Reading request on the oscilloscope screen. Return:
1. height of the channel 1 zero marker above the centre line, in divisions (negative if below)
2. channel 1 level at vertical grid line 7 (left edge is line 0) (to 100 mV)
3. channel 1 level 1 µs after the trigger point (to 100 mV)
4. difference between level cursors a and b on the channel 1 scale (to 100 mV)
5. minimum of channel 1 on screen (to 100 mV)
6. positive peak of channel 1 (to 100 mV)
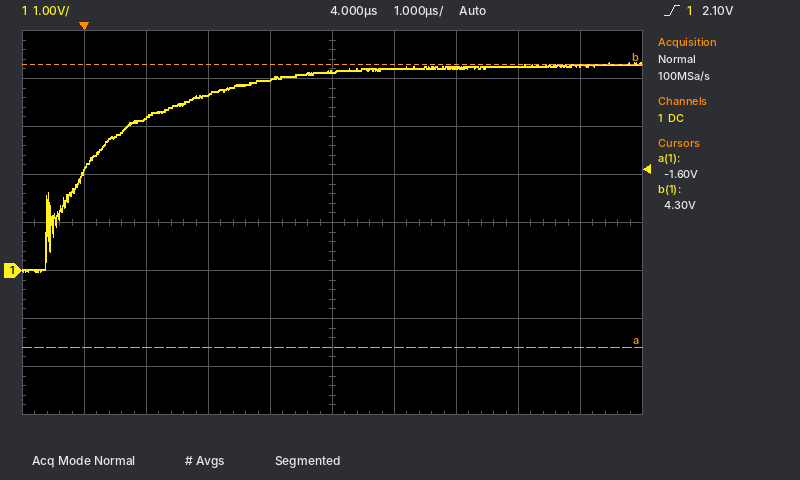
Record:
-1.0 div
4.2 V
3.2 V
5.9 V
0.0 V
4.3 V
